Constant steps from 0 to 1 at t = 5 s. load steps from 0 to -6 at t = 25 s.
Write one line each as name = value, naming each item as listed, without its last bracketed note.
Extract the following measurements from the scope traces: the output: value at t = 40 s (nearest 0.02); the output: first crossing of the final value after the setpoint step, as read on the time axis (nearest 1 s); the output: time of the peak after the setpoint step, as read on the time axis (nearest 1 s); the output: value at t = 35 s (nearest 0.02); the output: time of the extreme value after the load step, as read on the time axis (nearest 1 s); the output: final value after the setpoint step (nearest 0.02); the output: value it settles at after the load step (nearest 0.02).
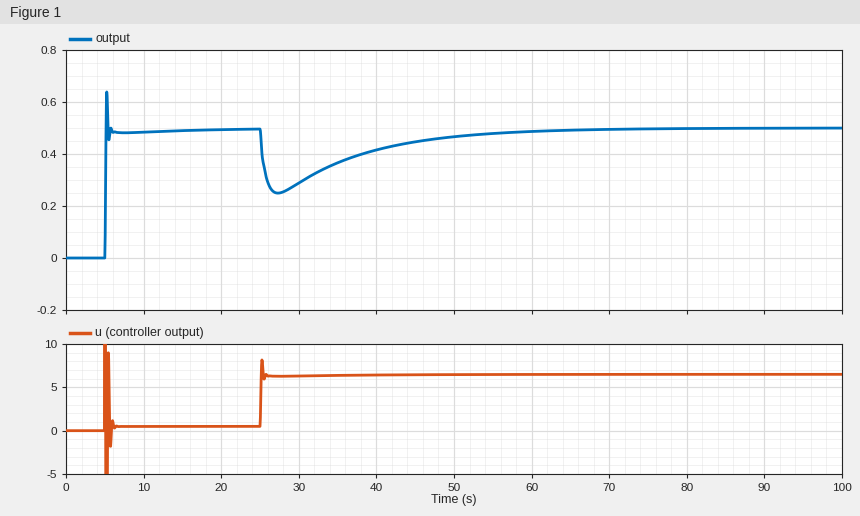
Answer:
the output: value at t = 40 s = 0.42
the output: first crossing of the final value after the setpoint step, as read on the time axis = 5 s
the output: time of the peak after the setpoint step, as read on the time axis = 5 s
the output: value at t = 35 s = 0.36
the output: time of the extreme value after the load step, as read on the time axis = 27 s
the output: final value after the setpoint step = 0.50
the output: value it settles at after the load step = 0.50
